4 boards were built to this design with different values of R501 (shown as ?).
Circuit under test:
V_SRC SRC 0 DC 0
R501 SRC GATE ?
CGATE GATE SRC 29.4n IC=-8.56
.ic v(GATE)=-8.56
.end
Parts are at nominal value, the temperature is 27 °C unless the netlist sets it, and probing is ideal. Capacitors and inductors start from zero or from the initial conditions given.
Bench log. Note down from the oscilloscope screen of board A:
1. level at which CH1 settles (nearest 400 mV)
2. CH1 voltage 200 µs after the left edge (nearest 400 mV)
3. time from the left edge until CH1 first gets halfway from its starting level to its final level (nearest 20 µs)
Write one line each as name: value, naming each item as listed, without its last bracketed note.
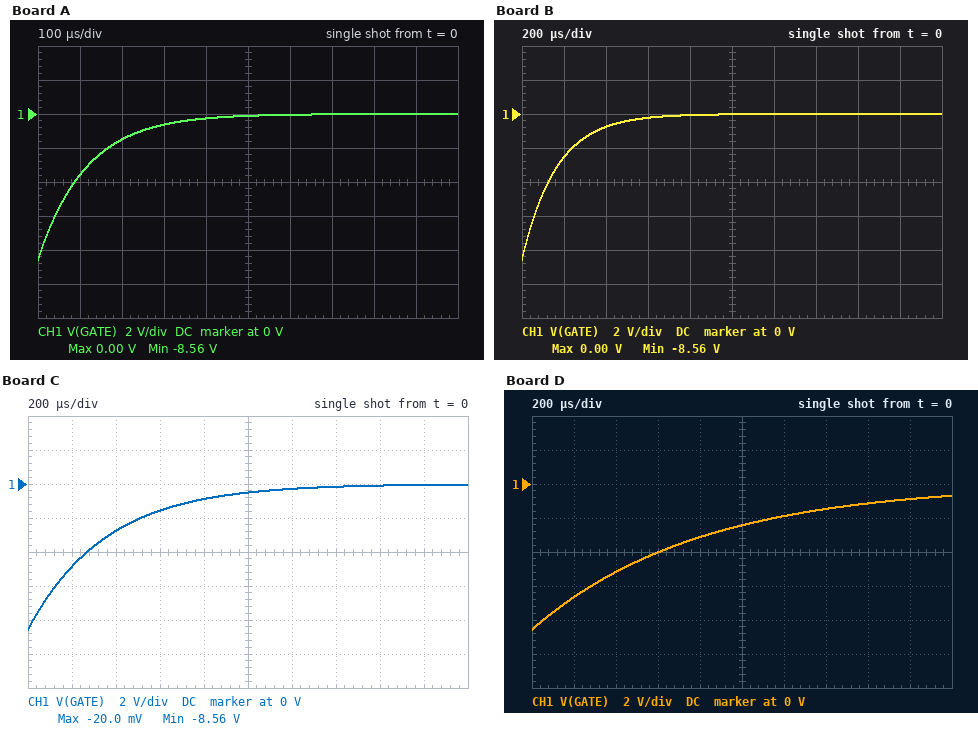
level at which CH1 settles: 0 V
CH1 voltage 200 µs after the left edge: -1.6 V
time from the left edge until CH1 first gets halfway from its starting level to its final level: 80 µs
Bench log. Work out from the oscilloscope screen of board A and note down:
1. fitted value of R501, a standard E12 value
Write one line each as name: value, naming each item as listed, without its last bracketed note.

fitted value of R501, a standard E12 value: 3.9 kΩ
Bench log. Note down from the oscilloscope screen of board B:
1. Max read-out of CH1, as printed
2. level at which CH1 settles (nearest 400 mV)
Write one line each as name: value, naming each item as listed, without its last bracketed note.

Max read-out of CH1, as printed: 0.00 V
level at which CH1 settles: 0 V
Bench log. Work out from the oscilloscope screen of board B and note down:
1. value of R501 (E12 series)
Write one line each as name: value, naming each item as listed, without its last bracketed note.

value of R501: 5.6 kΩ
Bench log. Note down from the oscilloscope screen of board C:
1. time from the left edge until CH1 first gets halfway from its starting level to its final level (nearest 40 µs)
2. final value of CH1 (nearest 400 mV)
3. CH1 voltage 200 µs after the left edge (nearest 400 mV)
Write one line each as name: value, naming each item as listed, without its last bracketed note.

time from the left edge until CH1 first gets halfway from its starting level to its final level: 240 µs
final value of CH1: 0 V
CH1 voltage 200 µs after the left edge: -4.8 V
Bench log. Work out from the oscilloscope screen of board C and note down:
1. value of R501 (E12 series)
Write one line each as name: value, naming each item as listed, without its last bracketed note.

value of R501: 12 kΩ
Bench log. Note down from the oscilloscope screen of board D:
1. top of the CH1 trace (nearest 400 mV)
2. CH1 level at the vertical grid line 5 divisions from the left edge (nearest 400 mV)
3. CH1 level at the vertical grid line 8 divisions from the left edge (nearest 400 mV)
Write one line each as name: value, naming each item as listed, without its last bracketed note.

top of the CH1 trace: -800 mV
CH1 level at the vertical grid line 5 divisions from the left edge: -2.4 V
CH1 level at the vertical grid line 8 divisions from the left edge: -1.2 V
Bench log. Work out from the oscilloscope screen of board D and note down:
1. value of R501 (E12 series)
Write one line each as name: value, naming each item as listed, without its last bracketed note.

value of R501: 27 kΩ
